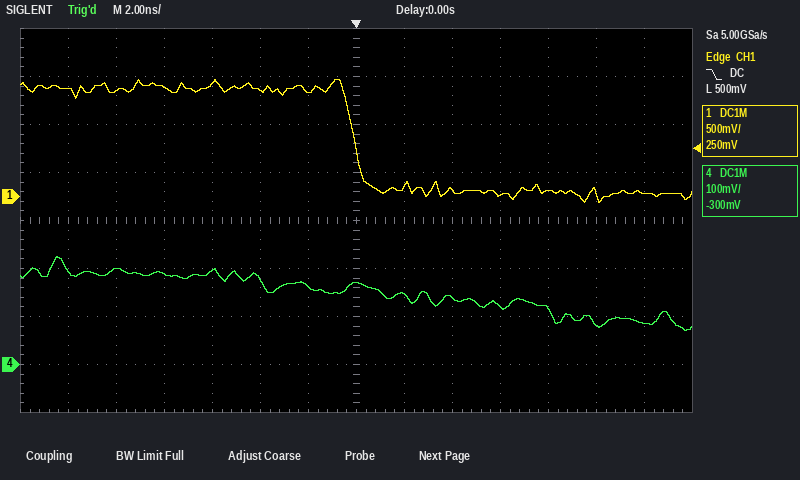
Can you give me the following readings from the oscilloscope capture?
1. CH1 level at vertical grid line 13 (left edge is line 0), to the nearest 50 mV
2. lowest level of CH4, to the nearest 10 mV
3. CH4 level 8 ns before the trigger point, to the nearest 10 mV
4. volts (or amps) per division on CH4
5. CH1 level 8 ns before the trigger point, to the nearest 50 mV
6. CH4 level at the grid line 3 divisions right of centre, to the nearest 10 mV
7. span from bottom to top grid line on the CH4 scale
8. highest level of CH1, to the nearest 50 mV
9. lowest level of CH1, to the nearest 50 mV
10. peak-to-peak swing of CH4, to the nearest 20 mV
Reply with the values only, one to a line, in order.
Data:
50 mV
70 mV
190 mV
100 mV
1.15 V
120 mV
800 mV
1.20 V
-50 mV
160 mV
